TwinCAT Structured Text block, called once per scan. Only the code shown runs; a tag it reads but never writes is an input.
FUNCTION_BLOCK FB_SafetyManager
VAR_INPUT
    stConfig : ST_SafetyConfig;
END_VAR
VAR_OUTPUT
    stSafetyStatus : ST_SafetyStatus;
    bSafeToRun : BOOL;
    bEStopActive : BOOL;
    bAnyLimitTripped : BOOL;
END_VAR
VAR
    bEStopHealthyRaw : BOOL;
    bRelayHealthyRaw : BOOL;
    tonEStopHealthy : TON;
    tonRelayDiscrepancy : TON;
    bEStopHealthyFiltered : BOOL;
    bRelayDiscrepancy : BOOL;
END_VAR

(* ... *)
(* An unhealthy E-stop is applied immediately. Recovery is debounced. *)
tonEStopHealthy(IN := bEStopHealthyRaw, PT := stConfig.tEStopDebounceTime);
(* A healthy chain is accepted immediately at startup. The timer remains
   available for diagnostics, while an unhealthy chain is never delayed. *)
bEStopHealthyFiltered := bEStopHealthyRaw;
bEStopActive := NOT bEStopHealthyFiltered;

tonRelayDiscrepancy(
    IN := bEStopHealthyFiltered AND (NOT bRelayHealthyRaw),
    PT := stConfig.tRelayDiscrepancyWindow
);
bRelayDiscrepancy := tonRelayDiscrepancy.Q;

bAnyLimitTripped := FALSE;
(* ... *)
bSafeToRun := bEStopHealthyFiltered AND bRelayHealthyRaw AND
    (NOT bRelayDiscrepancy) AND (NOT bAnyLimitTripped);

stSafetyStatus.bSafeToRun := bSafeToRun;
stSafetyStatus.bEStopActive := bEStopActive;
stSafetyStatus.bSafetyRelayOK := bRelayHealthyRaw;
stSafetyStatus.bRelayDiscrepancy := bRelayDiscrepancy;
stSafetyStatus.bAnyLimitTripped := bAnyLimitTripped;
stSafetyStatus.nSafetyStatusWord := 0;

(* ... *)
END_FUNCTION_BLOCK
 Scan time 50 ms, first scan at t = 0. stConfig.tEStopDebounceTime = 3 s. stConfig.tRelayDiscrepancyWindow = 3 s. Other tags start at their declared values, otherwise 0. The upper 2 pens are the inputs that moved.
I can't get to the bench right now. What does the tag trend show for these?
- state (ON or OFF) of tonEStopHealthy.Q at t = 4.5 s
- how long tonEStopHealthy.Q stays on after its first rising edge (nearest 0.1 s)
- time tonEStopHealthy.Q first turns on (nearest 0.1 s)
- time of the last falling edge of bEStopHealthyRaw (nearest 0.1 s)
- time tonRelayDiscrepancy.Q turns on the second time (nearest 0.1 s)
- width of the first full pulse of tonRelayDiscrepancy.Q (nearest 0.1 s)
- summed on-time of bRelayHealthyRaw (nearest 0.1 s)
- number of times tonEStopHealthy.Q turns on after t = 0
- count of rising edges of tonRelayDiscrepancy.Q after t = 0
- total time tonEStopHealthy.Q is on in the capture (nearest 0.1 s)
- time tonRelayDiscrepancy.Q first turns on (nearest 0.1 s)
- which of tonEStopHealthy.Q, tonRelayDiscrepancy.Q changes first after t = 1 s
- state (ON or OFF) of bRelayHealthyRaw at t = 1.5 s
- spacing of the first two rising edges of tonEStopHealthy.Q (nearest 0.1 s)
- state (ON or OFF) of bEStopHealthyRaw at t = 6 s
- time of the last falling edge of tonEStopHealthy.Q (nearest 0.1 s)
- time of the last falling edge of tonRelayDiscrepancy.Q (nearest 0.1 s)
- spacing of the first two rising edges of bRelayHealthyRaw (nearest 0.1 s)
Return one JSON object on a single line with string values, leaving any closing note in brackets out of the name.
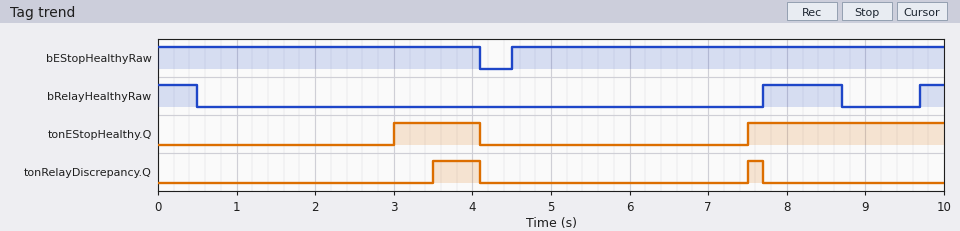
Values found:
{"state (ON or OFF) of tonEStopHealthy.Q at t = 4.5 s": "OFF", "how long tonEStopHealthy.Q stays on after its first rising edge": "1.1 s", "time tonEStopHealthy.Q first turns on": "3.0 s", "time of the last falling edge of bEStopHealthyRaw": "4.1 s", "time tonRelayDiscrepancy.Q turns on the second time": "7.5 s", "width of the first full pulse of tonRelayDiscrepancy.Q": "0.6 s", "summed on-time of bRelayHealthyRaw": "1.8 s", "number of times tonEStopHealthy.Q turns on after t = 0": "2", "count of rising edges of tonRelayDiscrepancy.Q after t = 0": "2", "total time tonEStopHealthy.Q is on in the capture": "3.6 s", "time tonRelayDiscrepancy.Q first turns on": "3.5 s", "which of tonEStopHealthy.Q, tonRelayDiscrepancy.Q changes first after t = 1 s": "tonEStopHealthy.Q", "state (ON or OFF) of bRelayHealthyRaw at t = 1.5 s": "OFF", "spacing of the first two rising edges of tonEStopHealthy.Q": "4.5 s", "state (ON or OFF) of bEStopHealthyRaw at t = 6 s": "ON", "time of the last falling edge of tonEStopHealthy.Q": "4.1 s", "time of the last falling edge of tonRelayDiscrepancy.Q": "7.7 s", "spacing of the first two rising edges of bRelayHealthyRaw": "2.0 s"}
